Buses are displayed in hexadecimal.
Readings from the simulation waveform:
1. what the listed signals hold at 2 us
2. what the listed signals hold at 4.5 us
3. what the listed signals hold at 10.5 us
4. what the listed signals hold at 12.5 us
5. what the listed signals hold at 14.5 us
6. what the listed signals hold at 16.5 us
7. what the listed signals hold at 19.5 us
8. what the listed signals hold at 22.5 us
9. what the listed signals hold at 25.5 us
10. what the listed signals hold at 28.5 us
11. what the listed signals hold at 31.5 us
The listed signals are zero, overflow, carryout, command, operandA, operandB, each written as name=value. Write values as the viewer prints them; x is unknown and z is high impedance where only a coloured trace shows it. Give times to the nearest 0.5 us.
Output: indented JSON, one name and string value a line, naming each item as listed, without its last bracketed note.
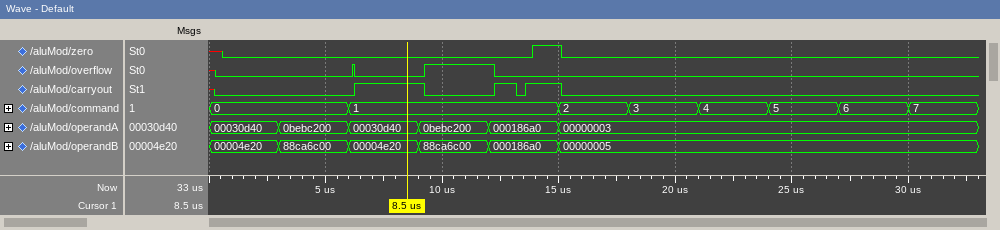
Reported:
{
  "what the listed signals hold at 2 us": "zero=0, overflow=0, carryout=0, command=0, operandA=00030d40, operandB=00004e20",
  "what the listed signals hold at 4.5 us": "zero=0, overflow=0, carryout=0, command=0, operandA=0bebc200, operandB=88ca6c00",
  "what the listed signals hold at 10.5 us": "zero=0, overflow=1, carryout=0, command=1, operandA=0bebc200, operandB=88ca6c00",
  "what the listed signals hold at 12.5 us": "zero=0, overflow=0, carryout=1, command=1, operandA=000186a0, operandB=000186a0",
  "what the listed signals hold at 14.5 us": "zero=1, overflow=0, carryout=1, command=1, operandA=000186a0, operandB=000186a0",
  "what the listed signals hold at 16.5 us": "zero=0, overflow=0, carryout=0, command=2, operandA=00000003, operandB=00000005",
  "what the listed signals hold at 19.5 us": "zero=0, overflow=0, carryout=0, command=3, operandA=00000003, operandB=00000005",
  "what the listed signals hold at 22.5 us": "zero=0, overflow=0, carryout=0, command=4, operandA=00000003, operandB=00000005",
  "what the listed signals hold at 25.5 us": "zero=0, overflow=0, carryout=0, command=5, operandA=00000003, operandB=00000005",
  "what the listed signals hold at 28.5 us": "zero=0, overflow=0, carryout=0, command=6, operandA=00000003, operandB=00000005",
  "what the listed signals hold at 31.5 us": "zero=0, overflow=0, carryout=0, command=7, operandA=00000003, operandB=00000005"
}
